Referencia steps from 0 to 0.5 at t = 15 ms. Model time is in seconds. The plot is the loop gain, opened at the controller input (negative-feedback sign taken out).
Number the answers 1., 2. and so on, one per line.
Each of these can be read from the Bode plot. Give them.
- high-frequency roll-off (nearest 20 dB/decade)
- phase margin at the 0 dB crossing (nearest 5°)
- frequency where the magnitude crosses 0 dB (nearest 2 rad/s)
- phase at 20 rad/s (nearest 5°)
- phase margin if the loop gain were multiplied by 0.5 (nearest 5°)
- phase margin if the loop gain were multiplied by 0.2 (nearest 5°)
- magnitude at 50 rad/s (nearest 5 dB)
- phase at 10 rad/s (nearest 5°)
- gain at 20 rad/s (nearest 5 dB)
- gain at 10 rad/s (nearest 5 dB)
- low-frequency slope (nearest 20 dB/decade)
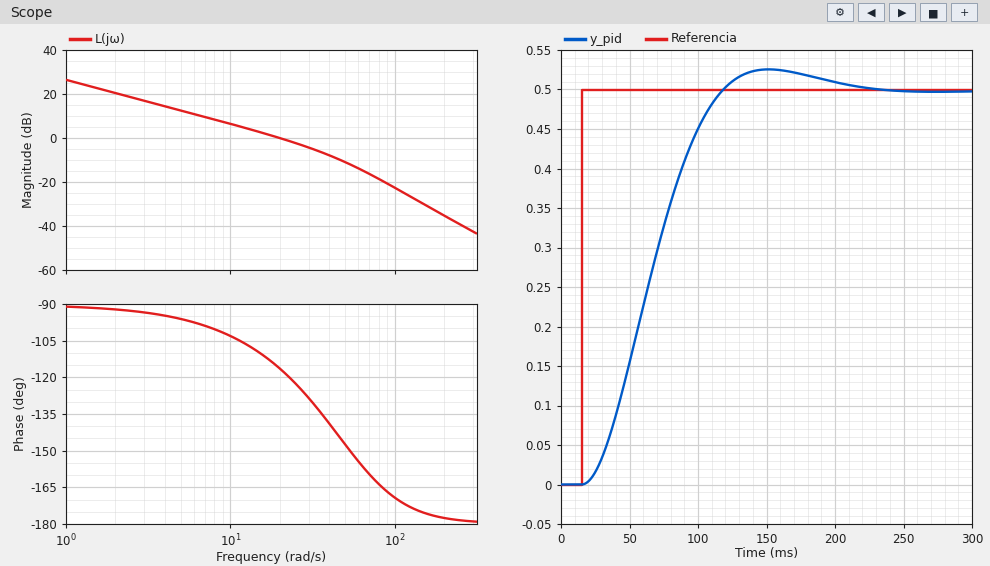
1. -40 dB/decade
2. 65°
3. 20 rad/s
4. -115°
5. 75°
6. 85°
7. -10 dB
8. -105°
9. 0 dB
10. 5 dB
11. -20 dB/decade
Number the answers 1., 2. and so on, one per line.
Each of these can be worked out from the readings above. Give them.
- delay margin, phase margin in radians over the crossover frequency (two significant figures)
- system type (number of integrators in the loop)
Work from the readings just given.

1. 0.057 s
2. 1
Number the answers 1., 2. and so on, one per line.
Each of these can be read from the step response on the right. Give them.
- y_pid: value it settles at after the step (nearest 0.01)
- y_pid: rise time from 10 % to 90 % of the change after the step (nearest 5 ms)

1. 0.50
2. 65 ms
